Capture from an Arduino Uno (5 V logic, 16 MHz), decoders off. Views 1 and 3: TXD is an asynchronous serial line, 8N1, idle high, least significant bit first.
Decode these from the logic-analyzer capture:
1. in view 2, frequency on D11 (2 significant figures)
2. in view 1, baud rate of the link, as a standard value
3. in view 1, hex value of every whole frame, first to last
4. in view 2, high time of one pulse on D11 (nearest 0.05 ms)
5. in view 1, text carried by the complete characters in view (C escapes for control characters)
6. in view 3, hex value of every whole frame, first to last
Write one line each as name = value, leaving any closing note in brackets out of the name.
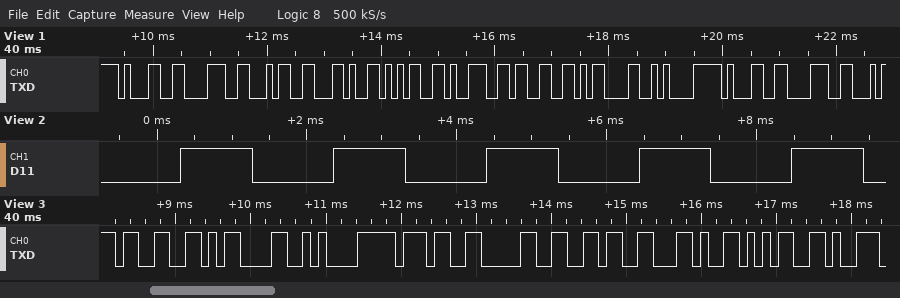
in view 2, frequency on D11 = 490 Hz
in view 1, baud rate of the link, as a standard value = 9600 baud
in view 1, hex value of every whole frame, first to last = 31 38 34 2C 35 39 33 0D 0A 31 38
in view 2, high time of one pulse on D11 = 0.95 ms
in view 1, text carried by the complete characters in view = "184,593\r\n18"
in view 3, hex value of every whole frame, first to last = 0x33 0x0D 0x0A 0x37 0x30 0x36 0x2C 0x35
